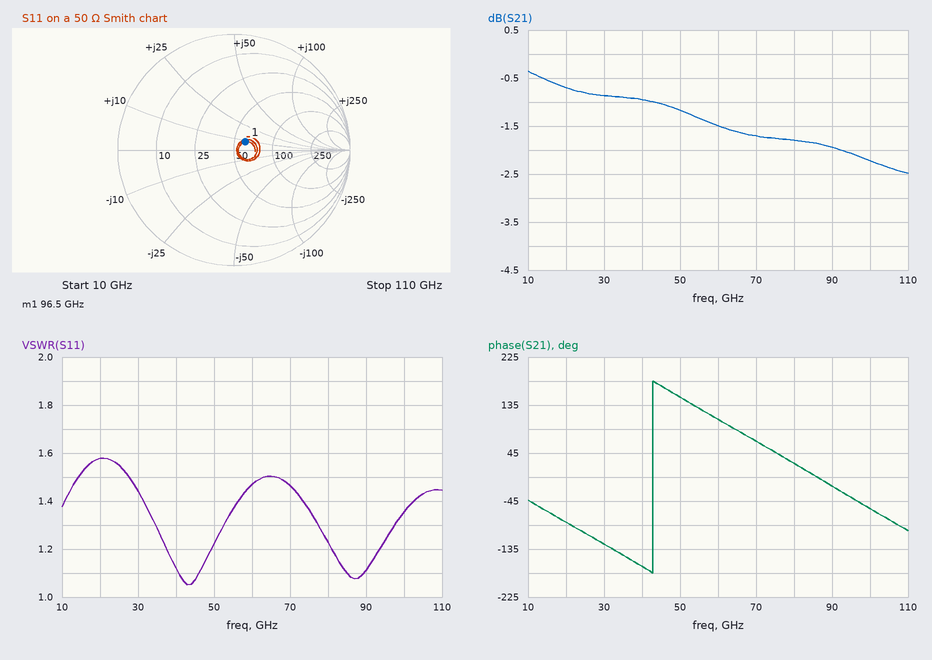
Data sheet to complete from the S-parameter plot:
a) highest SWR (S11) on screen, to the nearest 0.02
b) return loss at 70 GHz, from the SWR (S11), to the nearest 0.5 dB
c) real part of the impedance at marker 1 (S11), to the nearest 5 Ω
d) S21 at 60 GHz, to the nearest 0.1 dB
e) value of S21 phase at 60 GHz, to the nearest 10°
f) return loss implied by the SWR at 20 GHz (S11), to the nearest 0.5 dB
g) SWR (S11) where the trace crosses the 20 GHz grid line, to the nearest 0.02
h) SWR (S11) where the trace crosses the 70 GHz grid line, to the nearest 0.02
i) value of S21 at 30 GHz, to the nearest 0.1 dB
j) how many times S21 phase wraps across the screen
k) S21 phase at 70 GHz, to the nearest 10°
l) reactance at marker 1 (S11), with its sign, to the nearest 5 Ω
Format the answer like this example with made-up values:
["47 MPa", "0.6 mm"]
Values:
["1.58", "14.5 dB", "60 Ω", "-1.5 dB", "110°", "13.0 dB", "1.58", "1.46", "-0.9 dB", "1", "70°", "+10 Ω"]
